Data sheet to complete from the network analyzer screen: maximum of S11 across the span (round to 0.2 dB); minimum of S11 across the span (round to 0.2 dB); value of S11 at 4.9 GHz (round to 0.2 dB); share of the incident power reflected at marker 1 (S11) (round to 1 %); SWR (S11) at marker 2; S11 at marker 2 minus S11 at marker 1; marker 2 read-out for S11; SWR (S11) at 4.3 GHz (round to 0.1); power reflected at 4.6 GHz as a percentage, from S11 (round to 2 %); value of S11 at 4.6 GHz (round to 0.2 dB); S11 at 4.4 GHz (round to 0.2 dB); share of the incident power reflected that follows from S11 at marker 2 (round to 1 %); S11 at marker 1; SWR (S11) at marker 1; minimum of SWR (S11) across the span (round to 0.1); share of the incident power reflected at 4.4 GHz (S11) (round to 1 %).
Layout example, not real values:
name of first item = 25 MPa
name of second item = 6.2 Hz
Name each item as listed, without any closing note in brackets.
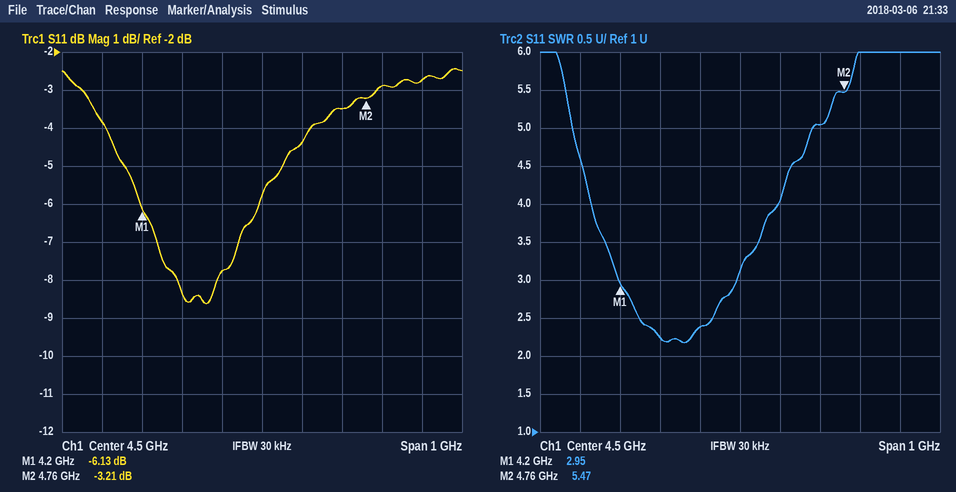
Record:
maximum of S11 across the span = -2.4 dB
minimum of S11 across the span = -8.6 dB
value of S11 at 4.9 GHz = -2.8 dB
share of the incident power reflected at marker 1 (S11) = 24 %
SWR (S11) at marker 2 = 5.47
S11 at marker 2 minus S11 at marker 1 = 2.92 dB
marker 2 read-out for S11 = -3.21 dB
SWR (S11) at 4.3 GHz = 2.2
power reflected at 4.6 GHz as a percentage, from S11 = 36 %
value of S11 at 4.6 GHz = -4.4 dB
S11 at 4.4 GHz = -7.8 dB
share of the incident power reflected that follows from S11 at marker 2 = 48 %
S11 at marker 1 = -6.13 dB
SWR (S11) at marker 1 = 2.95
minimum of SWR (S11) across the span = 2.2
share of the incident power reflected at 4.4 GHz (S11) = 17 %
